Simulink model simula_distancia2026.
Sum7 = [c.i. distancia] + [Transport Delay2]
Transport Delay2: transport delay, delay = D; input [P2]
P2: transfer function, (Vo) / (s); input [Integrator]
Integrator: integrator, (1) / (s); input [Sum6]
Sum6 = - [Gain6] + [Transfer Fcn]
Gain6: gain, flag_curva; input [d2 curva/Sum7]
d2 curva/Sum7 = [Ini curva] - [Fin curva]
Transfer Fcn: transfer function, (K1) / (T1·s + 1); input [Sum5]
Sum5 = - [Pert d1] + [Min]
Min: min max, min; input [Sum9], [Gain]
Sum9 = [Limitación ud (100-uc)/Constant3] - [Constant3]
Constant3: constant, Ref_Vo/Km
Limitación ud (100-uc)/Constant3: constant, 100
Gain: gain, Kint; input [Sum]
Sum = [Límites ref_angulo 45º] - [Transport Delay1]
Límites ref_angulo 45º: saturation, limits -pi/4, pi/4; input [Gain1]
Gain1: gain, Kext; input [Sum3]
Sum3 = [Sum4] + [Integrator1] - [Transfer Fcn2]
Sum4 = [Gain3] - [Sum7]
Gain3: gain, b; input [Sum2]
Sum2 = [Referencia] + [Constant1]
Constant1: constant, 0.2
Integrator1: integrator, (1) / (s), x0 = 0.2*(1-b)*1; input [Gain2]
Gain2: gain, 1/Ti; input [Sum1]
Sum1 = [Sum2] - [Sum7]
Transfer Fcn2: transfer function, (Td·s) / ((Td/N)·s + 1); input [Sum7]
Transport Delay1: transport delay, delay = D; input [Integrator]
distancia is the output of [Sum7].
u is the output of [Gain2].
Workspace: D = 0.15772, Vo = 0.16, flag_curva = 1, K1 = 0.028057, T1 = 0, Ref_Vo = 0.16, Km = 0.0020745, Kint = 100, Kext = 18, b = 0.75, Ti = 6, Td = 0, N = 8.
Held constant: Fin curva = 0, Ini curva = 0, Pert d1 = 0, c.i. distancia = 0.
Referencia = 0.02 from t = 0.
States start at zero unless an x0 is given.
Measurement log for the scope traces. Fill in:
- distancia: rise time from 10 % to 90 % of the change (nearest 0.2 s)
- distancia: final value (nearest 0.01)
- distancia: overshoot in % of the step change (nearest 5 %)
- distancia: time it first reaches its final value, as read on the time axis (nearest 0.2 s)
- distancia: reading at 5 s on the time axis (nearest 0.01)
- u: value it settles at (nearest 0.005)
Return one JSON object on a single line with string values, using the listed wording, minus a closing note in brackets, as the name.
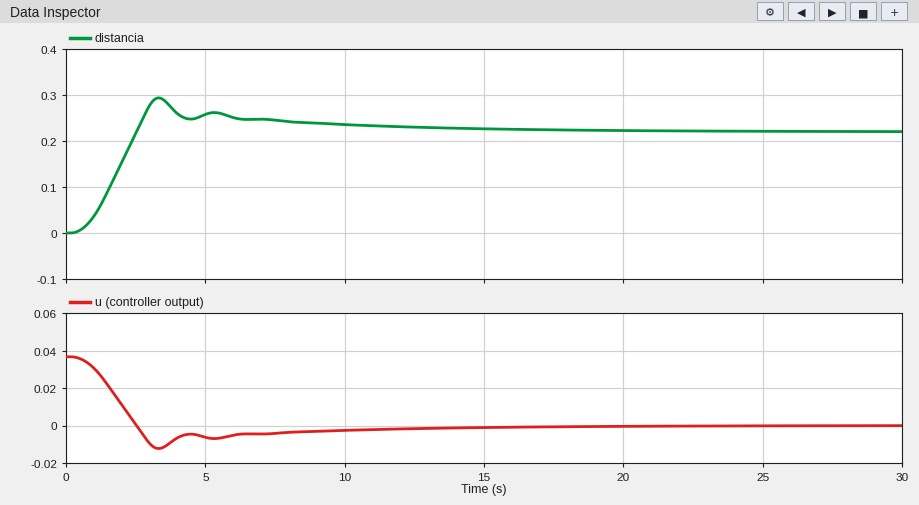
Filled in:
{"distancia: rise time from 10 % to 90 % of the change": "1.6 s", "distancia: final value": "0.22", "distancia: overshoot in % of the step change": "35 %", "distancia: time it first reaches its final value, as read on the time axis": "2.6 s", "distancia: reading at 5 s on the time axis": "0.26", "u: value it settles at": "0.000"}
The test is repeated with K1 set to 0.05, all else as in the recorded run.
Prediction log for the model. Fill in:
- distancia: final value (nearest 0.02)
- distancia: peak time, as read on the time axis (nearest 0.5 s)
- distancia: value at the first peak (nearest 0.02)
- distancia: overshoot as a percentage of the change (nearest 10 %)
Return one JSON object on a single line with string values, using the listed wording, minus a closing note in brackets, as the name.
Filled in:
{"distancia: final value": "0.22", "distancia: peak time, as read on the time axis": "3.0 s", "distancia: value at the first peak": "0.28", "distancia: overshoot as a percentage of the change": "20 %"}
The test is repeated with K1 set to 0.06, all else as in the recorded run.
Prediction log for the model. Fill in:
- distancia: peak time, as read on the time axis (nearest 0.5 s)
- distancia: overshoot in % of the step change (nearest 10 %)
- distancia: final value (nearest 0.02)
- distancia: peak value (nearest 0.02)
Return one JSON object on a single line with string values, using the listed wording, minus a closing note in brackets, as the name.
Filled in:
{"distancia: peak time, as read on the time axis": "2.5 s", "distancia: overshoot in % of the step change": "20 %", "distancia: final value": "0.22", "distancia: peak value": "0.26"}
